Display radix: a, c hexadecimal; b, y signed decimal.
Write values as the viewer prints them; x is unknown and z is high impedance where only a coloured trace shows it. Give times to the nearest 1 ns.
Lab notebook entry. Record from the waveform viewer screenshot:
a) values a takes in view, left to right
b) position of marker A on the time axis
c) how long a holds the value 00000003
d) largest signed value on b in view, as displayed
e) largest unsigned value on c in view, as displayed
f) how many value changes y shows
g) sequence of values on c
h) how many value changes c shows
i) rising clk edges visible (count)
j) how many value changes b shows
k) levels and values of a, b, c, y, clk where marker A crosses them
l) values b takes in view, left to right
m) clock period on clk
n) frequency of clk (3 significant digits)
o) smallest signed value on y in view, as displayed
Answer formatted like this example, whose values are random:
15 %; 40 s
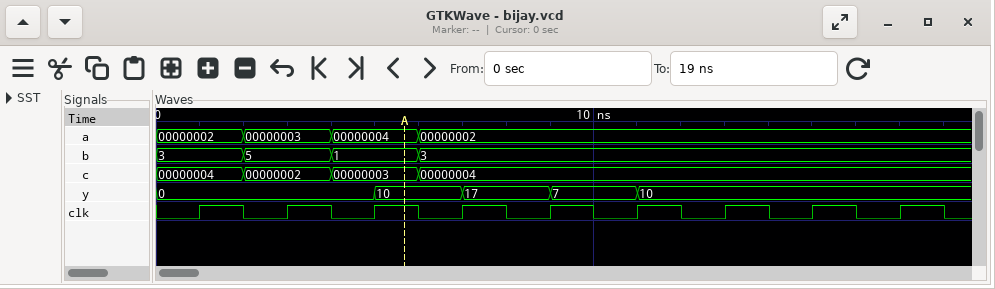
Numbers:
00000002, 00000003, 00000004, 00000002; 6 ns; 2 ns; 5; 00000004; 4; 00000004, 00000002, 00000003, 00000004; 3; 9; 3; a=00000004, b=1, c=00000003, y=10, clk=1; 3, 5, 1, 3; 2 ns; 500 MHz; 0
